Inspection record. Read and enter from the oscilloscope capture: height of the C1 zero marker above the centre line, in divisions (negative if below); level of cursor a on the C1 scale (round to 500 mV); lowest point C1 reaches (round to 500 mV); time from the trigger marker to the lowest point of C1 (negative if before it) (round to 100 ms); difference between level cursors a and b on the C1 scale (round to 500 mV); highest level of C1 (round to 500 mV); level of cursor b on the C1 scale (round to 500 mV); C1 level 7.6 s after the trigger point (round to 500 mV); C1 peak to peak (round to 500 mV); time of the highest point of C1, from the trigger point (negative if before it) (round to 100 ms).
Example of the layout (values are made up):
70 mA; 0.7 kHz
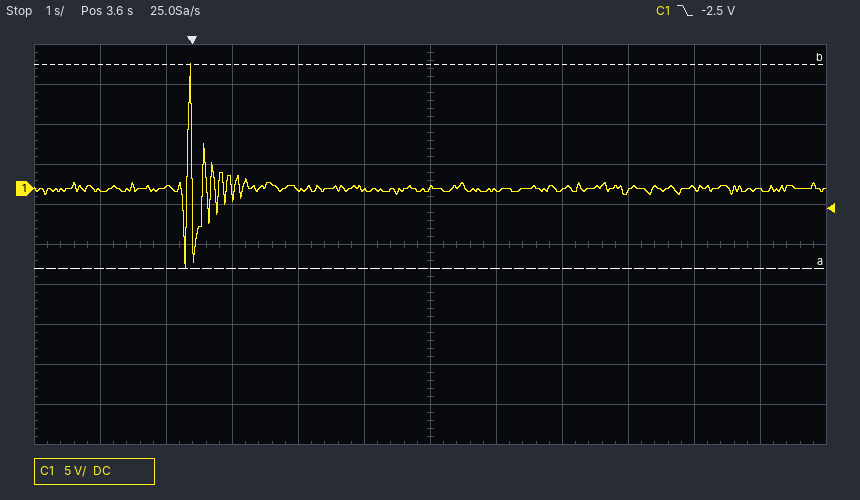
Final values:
+1.4 div; -10.0 V; -10.0 V; -100 ms; 25.5 V; 15.5 V; 15.5 V; 0.0 V; 25.5 V; 0.0 s
